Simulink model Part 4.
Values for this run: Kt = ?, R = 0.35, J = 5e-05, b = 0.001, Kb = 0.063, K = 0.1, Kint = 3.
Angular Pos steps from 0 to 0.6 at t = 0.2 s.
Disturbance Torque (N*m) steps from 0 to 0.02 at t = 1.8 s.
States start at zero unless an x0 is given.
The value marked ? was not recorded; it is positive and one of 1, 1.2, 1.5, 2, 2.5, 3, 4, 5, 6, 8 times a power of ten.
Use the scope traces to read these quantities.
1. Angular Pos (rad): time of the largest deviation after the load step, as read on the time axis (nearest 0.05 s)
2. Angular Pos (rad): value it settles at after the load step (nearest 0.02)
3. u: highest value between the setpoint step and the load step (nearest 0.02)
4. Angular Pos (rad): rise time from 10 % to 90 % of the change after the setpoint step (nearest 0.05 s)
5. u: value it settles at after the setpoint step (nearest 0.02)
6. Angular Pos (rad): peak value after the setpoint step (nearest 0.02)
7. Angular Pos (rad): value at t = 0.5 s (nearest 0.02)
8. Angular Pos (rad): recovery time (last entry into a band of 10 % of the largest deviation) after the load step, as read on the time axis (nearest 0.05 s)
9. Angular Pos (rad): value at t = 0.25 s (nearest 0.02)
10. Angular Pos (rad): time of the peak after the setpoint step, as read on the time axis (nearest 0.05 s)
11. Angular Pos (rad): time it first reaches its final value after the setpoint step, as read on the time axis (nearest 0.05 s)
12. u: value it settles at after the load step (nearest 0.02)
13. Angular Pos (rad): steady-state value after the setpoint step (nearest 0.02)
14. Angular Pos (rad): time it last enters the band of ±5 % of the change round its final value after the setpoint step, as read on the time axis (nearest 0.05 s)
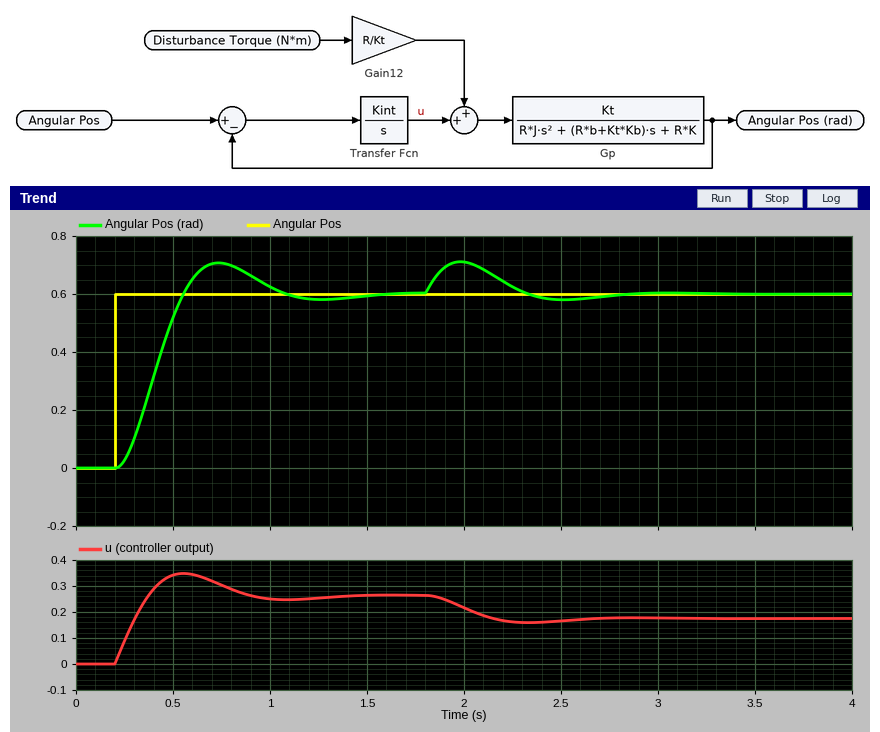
2.00 s
0.60
0.34
0.25 s
0.26
0.70
0.52
2.70 s
0.02
0.75 s
0.55 s
0.18
0.60
1.00 s
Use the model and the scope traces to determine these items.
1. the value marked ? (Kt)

0.08
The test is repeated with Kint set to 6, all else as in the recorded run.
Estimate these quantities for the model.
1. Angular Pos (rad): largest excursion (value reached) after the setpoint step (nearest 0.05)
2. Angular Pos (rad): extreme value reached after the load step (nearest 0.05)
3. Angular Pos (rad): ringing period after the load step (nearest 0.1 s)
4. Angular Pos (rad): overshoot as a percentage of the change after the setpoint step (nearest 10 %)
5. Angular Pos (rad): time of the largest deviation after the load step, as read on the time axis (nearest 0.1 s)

0.80
0.70
0.7 s
30 %
1.9 s
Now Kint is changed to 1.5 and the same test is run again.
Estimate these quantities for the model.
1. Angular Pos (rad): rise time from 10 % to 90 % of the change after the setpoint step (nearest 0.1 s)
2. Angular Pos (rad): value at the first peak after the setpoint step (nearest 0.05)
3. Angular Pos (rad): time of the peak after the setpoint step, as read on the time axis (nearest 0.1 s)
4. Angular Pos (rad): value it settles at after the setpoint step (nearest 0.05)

0.4 s
0.65
1.1 s
0.60
